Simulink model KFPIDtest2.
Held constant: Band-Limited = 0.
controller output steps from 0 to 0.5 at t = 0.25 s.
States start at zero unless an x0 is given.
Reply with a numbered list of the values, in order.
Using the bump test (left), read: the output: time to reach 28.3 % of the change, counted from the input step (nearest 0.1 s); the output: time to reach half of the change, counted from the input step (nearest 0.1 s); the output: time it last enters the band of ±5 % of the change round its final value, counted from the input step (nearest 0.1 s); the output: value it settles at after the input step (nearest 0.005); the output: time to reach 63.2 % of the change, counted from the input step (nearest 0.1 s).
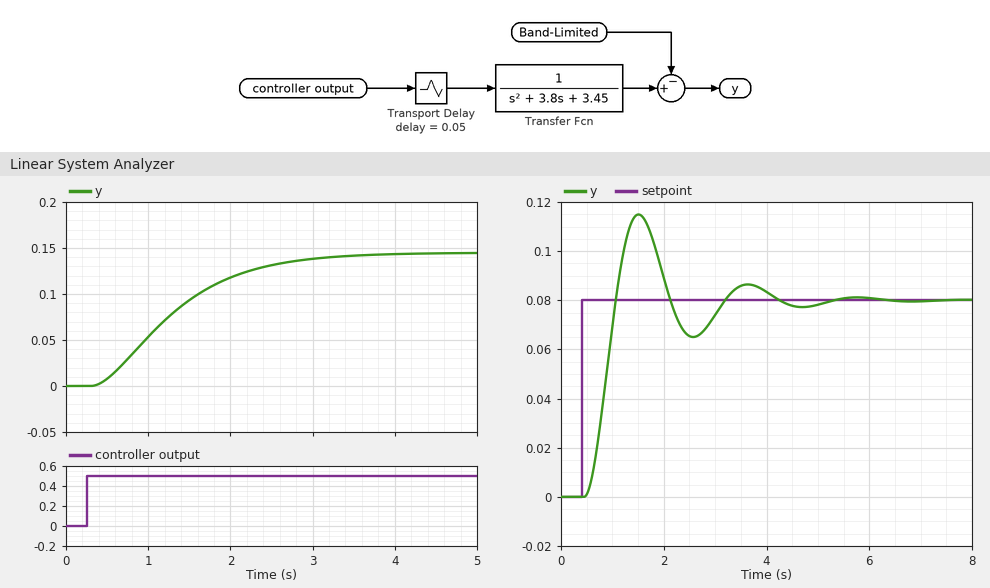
1. 0.6 s
2. 1.0 s
3. 2.7 s
4. 0.145
5. 1.2 s
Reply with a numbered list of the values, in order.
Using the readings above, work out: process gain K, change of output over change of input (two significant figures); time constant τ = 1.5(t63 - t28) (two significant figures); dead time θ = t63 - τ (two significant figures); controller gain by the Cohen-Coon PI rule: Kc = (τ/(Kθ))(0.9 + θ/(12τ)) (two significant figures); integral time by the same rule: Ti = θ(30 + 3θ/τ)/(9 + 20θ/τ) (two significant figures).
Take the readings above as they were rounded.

1. 0.29
2. 0.90 s
3. 0.30 s
4. 9.6
5. 0.59 s
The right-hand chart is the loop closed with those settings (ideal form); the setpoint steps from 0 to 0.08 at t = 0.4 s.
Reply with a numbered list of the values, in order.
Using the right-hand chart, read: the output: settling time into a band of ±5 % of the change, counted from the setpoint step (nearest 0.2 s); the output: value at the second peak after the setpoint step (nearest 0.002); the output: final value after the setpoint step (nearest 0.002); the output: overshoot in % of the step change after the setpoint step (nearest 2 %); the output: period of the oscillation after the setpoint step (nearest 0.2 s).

1. 3.6 s
2. 0.086
3. 0.080
4. 44 %
5. 2.2 s
